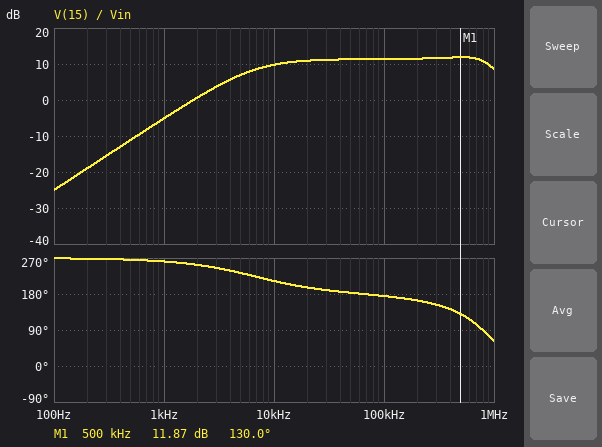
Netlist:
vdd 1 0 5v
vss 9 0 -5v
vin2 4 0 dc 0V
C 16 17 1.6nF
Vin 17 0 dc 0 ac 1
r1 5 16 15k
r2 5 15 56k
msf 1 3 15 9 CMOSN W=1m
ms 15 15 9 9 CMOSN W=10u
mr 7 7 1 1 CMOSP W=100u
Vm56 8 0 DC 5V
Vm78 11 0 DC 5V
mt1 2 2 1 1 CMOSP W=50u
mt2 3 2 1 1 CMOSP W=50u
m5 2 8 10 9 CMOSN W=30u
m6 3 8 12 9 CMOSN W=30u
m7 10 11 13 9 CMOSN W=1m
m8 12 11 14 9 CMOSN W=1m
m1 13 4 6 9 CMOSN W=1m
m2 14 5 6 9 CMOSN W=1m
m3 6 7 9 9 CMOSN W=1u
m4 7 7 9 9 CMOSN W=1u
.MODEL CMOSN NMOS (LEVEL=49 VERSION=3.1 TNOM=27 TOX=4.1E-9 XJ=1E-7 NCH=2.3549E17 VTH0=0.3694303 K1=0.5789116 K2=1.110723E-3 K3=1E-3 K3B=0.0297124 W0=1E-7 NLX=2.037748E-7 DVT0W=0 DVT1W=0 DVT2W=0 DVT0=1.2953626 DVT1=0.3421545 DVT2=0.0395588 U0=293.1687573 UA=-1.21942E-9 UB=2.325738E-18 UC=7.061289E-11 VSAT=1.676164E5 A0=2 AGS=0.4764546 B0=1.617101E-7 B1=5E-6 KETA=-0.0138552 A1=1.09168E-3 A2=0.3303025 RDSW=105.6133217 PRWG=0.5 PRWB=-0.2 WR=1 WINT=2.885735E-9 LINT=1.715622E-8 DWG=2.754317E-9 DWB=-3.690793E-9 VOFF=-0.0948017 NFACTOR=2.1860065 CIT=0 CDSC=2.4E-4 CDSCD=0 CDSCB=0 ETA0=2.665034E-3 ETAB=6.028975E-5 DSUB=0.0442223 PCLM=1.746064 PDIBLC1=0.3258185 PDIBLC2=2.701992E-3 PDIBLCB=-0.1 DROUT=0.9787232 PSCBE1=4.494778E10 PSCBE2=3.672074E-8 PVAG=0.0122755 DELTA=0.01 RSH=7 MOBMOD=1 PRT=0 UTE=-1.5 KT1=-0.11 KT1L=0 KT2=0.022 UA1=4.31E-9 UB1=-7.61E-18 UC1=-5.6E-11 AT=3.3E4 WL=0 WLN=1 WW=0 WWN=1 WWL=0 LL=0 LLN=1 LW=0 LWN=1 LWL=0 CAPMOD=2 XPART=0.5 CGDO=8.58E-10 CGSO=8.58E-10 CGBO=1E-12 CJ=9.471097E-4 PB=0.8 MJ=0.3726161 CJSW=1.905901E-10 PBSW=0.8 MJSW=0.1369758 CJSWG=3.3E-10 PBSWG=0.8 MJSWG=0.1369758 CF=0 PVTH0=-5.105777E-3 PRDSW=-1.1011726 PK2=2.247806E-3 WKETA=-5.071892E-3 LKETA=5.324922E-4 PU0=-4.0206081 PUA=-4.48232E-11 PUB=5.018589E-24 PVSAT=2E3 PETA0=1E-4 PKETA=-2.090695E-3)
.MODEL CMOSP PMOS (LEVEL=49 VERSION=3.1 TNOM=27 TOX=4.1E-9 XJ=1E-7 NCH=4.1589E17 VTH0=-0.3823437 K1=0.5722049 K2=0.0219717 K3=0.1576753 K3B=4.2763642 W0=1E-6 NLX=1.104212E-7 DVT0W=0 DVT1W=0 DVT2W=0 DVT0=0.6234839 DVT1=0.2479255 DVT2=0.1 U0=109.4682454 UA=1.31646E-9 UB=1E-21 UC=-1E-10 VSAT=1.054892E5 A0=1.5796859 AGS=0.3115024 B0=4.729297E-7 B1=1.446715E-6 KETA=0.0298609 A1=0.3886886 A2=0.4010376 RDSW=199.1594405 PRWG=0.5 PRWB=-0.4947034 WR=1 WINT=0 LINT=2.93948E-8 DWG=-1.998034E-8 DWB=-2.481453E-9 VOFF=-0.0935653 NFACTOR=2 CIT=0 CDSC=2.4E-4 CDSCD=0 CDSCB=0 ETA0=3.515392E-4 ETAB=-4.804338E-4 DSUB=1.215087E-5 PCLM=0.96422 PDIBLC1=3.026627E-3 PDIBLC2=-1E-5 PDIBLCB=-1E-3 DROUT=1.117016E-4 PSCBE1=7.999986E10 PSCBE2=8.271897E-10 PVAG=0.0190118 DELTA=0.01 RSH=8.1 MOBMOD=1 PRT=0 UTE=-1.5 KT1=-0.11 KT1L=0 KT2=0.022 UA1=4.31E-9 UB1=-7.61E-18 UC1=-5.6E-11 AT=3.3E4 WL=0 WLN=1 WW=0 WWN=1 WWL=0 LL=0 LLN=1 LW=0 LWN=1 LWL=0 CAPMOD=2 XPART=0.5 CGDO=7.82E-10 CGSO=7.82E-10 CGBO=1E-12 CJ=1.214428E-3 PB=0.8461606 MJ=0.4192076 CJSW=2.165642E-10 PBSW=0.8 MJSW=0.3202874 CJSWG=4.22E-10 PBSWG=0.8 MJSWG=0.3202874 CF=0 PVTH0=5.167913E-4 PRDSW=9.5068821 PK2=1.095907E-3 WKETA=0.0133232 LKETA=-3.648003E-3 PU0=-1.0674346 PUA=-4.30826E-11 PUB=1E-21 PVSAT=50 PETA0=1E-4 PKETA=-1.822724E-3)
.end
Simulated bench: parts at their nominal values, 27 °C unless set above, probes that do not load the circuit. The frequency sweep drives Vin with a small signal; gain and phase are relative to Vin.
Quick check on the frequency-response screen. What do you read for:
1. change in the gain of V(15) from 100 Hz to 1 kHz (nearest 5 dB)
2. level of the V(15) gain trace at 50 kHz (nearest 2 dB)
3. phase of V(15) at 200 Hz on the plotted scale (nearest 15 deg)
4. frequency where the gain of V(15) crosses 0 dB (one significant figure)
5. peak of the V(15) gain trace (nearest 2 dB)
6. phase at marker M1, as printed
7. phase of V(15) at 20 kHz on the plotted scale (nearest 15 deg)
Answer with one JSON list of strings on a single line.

["20 dB", "12 dB", "270 deg", "2 kHz", "12 dB", "130.0 deg", "195 deg"]
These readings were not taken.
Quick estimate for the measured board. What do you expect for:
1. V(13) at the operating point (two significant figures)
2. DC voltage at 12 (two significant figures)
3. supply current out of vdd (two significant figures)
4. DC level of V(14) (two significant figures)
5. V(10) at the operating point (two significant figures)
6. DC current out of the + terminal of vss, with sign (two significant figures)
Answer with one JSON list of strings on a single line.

["3.1 V", "1.5 V", "3.0 mA", "1.5 V", "3.1 V", "-3.0 mA"]
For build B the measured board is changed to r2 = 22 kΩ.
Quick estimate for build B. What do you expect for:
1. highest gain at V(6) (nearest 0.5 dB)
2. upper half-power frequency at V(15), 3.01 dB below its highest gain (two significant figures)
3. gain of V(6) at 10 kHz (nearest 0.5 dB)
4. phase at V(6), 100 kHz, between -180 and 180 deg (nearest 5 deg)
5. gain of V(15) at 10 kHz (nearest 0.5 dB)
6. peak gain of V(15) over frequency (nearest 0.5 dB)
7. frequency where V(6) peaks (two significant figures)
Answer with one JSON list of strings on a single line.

["-10.0 dB", "1.5 MHz", "-57.0 dB", "90 deg", "1.5 dB", "6.5 dB", "1.3 MHz"]
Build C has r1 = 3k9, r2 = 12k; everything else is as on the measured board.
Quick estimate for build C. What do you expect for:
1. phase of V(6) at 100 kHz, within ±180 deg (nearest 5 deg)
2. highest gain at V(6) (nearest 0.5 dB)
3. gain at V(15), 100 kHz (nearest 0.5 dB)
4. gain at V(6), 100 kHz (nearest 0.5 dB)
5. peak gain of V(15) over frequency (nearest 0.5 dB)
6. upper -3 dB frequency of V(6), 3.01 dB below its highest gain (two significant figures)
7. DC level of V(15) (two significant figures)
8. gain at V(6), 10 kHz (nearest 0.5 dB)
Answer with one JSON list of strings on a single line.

["100 deg", "-8.5 dB", "9.5 dB", "-29.5 dB", "10.0 dB", "3.7 MHz", "4.7 mV", "-57.5 dB"]
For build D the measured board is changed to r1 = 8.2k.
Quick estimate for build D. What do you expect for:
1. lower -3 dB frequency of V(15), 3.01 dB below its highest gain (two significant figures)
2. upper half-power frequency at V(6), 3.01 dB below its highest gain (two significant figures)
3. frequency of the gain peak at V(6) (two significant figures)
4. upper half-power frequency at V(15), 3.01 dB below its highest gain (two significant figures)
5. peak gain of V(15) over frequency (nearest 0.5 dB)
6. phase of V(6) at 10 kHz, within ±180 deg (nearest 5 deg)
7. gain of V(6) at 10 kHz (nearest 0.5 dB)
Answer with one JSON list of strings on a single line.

["12 kHz", "2.0 MHz", "880 kHz", "640 kHz", "16.5 dB", "120 deg", "-46.0 dB"]
